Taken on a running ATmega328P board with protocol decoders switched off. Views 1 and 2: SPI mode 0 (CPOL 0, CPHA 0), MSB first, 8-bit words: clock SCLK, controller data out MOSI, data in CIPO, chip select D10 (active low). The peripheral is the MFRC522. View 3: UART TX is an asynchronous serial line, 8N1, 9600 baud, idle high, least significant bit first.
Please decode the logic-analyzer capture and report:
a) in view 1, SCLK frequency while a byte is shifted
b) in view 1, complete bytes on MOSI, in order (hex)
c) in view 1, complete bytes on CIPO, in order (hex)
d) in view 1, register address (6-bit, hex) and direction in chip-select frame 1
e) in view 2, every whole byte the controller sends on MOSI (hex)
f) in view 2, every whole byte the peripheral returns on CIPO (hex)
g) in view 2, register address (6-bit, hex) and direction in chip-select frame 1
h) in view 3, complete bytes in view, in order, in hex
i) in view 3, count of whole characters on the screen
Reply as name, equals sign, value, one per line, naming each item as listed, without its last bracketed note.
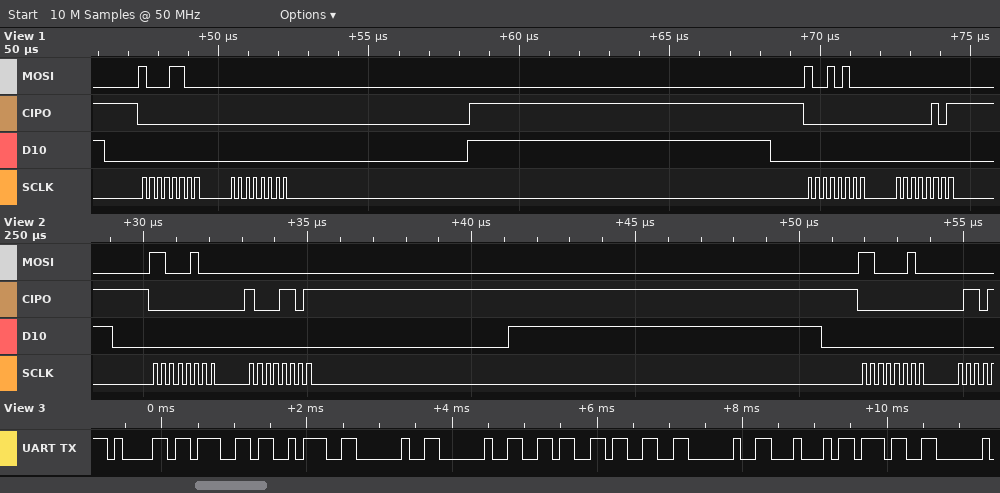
in view 1, SCLK frequency while a byte is shifted = 4 MHz
in view 1, complete bytes on MOSI, in order = 0x8C 0x00 0x94 0x00
in view 1, complete bytes on CIPO, in order = 0x00 0x00 0x00 0x05
in view 1, register address (6-bit, hex) and direction in chip-select frame 1 = 0x06 read
in view 2, every whole byte the controller sends on MOSI = C4 00 C2
in view 2, every whole byte the peripheral returns on CIPO = 00 8D 00
in view 2, register address (6-bit, hex) and direction in chip-select frame 1 = 0x22 read
in view 3, complete bytes in view, in order, in hex = 61 67 3A 20 20 36 33 20 44 37
in view 3, count of whole characters on the screen = 10
